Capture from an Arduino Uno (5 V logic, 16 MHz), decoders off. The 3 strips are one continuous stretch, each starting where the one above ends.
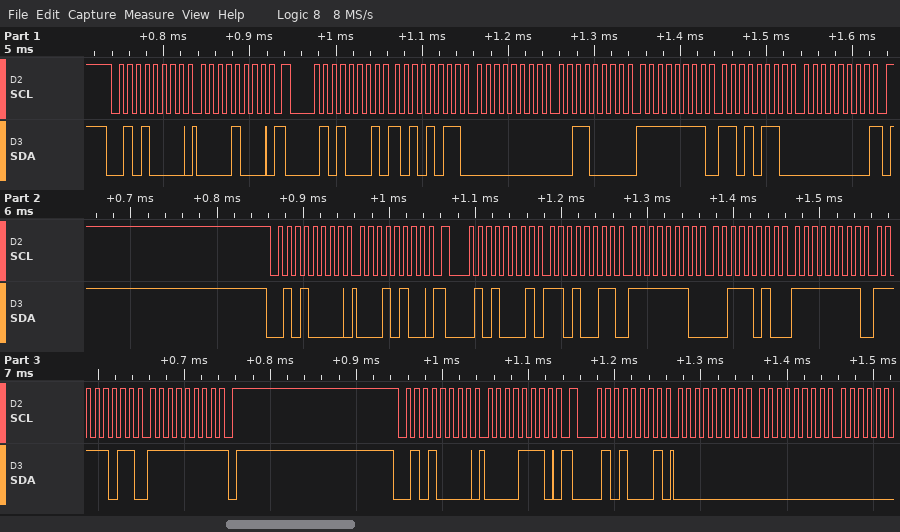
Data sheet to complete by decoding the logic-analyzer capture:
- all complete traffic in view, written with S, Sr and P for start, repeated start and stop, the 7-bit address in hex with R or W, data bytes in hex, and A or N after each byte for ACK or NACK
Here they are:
S 28W A 08 A Sr 28R A AB A 00 A 30 A FF A D6 A 00 N P S 28W A 14 A Sr 28R A D3 A FE A 3A A FF A FB A FF N P S 28W A 0E A Sr 28R A 00 A 00 A
